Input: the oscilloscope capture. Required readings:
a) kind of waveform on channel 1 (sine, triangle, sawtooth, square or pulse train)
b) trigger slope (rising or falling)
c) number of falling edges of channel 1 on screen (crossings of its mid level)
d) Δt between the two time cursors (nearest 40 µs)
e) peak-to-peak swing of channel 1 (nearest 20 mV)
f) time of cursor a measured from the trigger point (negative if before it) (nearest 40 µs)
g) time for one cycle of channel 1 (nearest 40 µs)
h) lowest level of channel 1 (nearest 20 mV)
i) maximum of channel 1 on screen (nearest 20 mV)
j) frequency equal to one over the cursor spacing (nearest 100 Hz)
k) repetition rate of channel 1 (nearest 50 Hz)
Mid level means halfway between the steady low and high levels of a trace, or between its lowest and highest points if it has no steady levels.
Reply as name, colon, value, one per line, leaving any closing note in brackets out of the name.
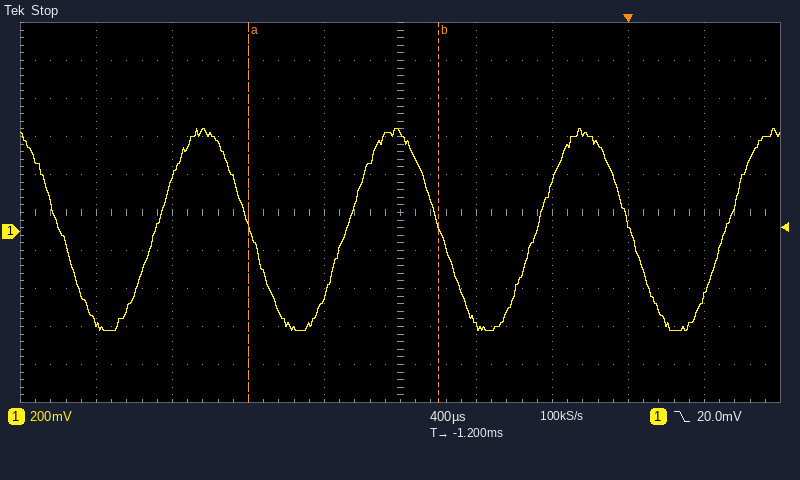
kind of waveform on channel 1: sine
trigger slope: falling
number of falling edges of channel 1 on screen: 4
Δt between the two time cursors: 1.00 ms
peak-to-peak swing of channel 1: 1.06 V
time of cursor a measured from the trigger point (negative if before it): -2.00 ms
time for one cycle of channel 1: 1.00 ms
lowest level of channel 1: -520 mV
maximum of channel 1 on screen: 540 mV
frequency equal to one over the cursor spacing: 1.0 kHz
repetition rate of channel 1: 1.00 kHz
